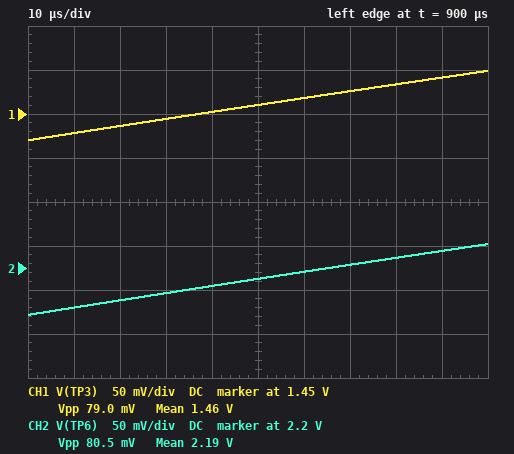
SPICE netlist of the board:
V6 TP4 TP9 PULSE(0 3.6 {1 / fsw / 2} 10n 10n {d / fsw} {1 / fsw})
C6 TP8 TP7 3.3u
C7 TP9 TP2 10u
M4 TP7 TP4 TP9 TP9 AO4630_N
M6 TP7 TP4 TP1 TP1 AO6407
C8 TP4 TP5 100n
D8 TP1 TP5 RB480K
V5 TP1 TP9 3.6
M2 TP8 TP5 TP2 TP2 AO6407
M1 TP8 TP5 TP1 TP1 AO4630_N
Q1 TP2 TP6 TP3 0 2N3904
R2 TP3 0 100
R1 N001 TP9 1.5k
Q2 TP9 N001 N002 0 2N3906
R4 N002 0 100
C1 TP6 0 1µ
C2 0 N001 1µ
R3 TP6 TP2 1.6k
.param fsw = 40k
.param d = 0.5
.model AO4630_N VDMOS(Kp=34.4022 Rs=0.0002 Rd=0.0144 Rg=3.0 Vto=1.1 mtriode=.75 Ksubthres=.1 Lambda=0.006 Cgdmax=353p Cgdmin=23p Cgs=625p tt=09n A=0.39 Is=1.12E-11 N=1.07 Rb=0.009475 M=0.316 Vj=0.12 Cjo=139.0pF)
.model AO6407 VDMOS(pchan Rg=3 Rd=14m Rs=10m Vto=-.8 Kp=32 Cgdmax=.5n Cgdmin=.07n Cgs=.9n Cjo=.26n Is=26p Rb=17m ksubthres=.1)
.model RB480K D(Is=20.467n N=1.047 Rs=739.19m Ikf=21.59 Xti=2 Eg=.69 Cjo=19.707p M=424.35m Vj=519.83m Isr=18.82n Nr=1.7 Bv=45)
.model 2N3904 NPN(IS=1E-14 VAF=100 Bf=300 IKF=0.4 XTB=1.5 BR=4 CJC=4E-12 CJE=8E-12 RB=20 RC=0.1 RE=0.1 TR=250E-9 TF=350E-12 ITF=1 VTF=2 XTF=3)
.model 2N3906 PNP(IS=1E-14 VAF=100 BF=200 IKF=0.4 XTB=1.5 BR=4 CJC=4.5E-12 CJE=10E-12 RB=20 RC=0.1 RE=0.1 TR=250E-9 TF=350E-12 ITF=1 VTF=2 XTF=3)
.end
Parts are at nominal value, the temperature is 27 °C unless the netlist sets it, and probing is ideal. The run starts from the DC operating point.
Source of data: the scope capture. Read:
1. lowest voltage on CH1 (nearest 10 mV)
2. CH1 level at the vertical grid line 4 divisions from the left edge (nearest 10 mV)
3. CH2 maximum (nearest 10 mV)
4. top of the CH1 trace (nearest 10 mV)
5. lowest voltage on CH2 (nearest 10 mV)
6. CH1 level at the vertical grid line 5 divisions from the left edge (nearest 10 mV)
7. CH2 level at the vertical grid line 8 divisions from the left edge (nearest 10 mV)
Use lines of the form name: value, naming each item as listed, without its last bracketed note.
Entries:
lowest voltage on CH1: 1.42 V
CH1 level at the vertical grid line 4 divisions from the left edge: 1.45 V
CH2 maximum: 2.23 V
top of the CH1 trace: 1.50 V
lowest voltage on CH2: 2.15 V
CH1 level at the vertical grid line 5 divisions from the left edge: 1.46 V
CH2 level at the vertical grid line 8 divisions from the left edge: 2.21 V
